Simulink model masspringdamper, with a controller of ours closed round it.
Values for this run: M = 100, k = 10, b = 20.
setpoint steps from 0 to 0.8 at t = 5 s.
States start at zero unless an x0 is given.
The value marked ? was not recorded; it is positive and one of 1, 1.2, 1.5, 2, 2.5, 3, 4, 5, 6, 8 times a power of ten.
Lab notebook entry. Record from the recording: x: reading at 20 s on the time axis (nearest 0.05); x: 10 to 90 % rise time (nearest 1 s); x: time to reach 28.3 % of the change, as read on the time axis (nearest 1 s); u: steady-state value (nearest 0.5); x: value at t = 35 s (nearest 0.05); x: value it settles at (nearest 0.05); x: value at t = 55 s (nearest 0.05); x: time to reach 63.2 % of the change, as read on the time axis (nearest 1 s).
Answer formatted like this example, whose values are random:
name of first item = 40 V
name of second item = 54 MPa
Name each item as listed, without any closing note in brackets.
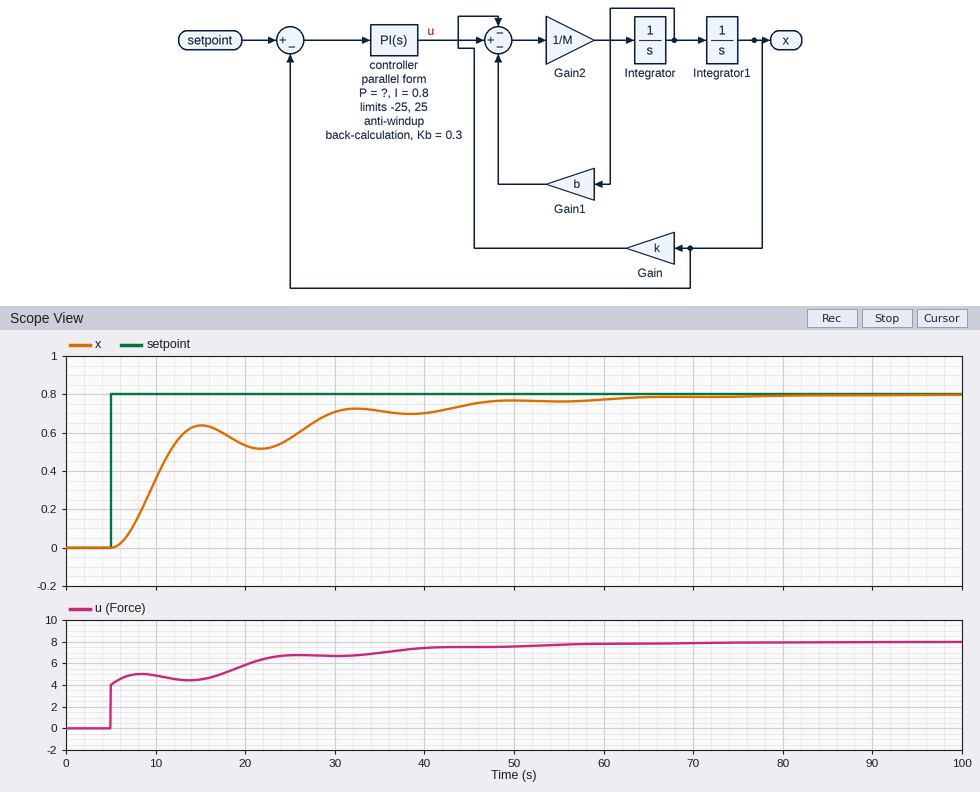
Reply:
x: reading at 20 s on the time axis = 0.55
x: 10 to 90 % rise time = 24 s
x: time to reach 28.3 % of the change, as read on the time axis = 9 s
u: steady-state value = 8.0
x: value at t = 35 s = 0.70
x: value it settles at = 0.80
x: value at t = 55 s = 0.75
x: time to reach 63.2 % of the change, as read on the time axis = 12 s
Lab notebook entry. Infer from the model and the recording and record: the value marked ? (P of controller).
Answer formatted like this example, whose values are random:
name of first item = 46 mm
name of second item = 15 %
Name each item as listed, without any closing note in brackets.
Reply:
the value marked ? = 5
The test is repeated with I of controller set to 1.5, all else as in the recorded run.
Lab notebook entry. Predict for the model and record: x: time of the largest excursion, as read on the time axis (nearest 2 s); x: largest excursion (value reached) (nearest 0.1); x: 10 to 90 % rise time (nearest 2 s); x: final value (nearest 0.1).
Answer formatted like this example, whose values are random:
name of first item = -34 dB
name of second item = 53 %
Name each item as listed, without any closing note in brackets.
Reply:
x: time of the largest excursion, as read on the time axis = 32 s
x: largest excursion (value reached) = 0.9
x: 10 to 90 % rise time = 6 s
x: final value = 0.8
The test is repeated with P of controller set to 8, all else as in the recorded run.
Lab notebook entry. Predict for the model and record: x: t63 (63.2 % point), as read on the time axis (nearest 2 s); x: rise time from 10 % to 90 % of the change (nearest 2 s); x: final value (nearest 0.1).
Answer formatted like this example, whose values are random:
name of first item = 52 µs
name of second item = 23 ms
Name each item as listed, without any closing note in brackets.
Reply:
x: t63 (63.2 % point), as read on the time axis = 10 s
x: rise time from 10 % to 90 % of the change = 34 s
x: final value = 0.8
